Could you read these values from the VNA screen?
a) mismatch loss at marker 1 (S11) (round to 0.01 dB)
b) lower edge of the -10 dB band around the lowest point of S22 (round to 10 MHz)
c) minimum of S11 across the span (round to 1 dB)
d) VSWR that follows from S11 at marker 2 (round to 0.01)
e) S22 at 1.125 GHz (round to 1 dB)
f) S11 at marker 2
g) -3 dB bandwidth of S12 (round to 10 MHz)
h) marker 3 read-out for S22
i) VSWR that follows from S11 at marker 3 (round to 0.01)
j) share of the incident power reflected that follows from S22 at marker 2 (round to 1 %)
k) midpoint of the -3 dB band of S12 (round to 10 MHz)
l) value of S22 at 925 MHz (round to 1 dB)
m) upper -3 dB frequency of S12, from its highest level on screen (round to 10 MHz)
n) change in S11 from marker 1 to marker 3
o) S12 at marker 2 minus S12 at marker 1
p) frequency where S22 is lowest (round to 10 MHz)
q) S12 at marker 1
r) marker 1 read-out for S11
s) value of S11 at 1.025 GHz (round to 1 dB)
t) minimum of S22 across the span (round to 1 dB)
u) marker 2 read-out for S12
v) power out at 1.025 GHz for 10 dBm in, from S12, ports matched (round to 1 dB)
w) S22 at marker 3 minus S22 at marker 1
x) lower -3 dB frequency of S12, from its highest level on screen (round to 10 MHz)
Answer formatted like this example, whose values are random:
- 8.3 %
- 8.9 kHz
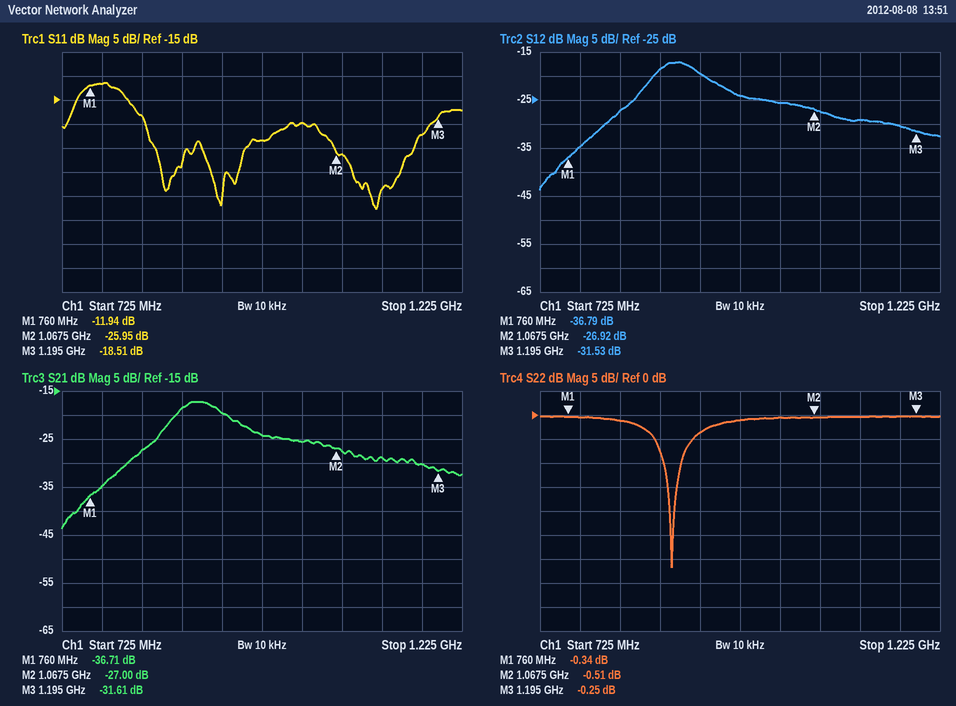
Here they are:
- 0.29 dB
- 880 MHz
- -38 dB
- 1.11
- 0 dB
- -25.95 dB
- 60 MHz
- -0.25 dB
- 1.27
- 89 %
- 900 MHz
- -4 dB
- 930 MHz
- -6.57 dB
- 9.87 dB
- 890 MHz
- -36.79 dB
- -11.94 dB
- -20 dB
- -32 dB
- -26.92 dB
- -16 dBm
- 0.09 dB
- 870 MHz
